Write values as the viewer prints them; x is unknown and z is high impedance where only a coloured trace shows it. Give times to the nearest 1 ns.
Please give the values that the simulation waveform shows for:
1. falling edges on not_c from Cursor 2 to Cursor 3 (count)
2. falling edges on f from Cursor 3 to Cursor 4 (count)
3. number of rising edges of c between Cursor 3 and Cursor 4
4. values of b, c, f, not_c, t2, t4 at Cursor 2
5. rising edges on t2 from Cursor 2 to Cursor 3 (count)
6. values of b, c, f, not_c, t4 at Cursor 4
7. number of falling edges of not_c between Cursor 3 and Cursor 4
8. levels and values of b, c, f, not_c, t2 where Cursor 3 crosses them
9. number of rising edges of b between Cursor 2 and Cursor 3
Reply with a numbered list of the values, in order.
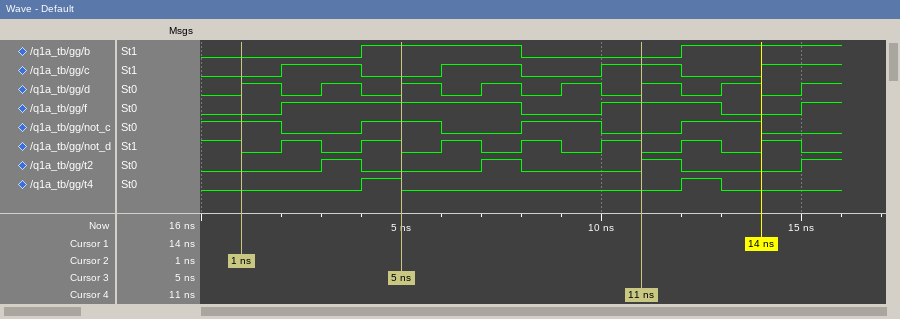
1. 1
2. 1
3. 2
4. b=0, c=0, f=0, not_c=1, t2=0, t4=0
5. 1
6. b=0, c=1, f=1, not_c=0, t4=0
7. 2
8. b=1, c=0, f=1, not_c=1, t2=0
9. 1
